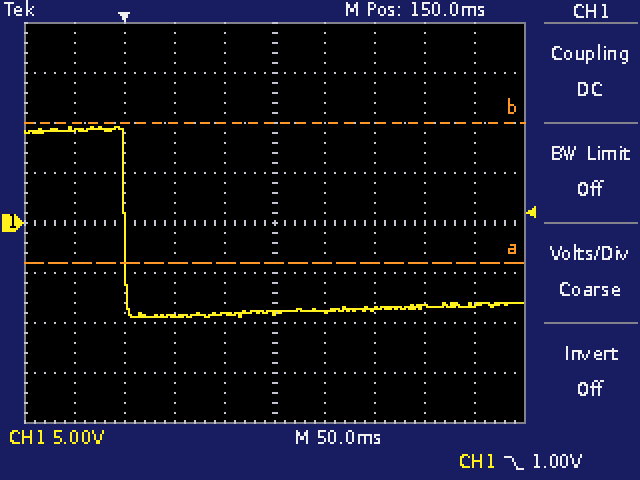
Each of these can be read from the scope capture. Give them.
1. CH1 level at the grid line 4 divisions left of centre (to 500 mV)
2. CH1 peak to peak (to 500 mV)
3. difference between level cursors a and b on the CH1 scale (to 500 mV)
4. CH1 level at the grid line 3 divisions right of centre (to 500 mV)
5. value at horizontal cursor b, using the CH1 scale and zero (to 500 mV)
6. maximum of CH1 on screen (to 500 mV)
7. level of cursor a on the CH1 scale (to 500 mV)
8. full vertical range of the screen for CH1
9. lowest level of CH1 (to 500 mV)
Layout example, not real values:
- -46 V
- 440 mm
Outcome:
- 9.5 V
- 19.0 V
- 14.0 V
- -8.5 V
- 10.0 V
- 9.5 V
- -4.0 V
- 40 V
- -9.5 V
